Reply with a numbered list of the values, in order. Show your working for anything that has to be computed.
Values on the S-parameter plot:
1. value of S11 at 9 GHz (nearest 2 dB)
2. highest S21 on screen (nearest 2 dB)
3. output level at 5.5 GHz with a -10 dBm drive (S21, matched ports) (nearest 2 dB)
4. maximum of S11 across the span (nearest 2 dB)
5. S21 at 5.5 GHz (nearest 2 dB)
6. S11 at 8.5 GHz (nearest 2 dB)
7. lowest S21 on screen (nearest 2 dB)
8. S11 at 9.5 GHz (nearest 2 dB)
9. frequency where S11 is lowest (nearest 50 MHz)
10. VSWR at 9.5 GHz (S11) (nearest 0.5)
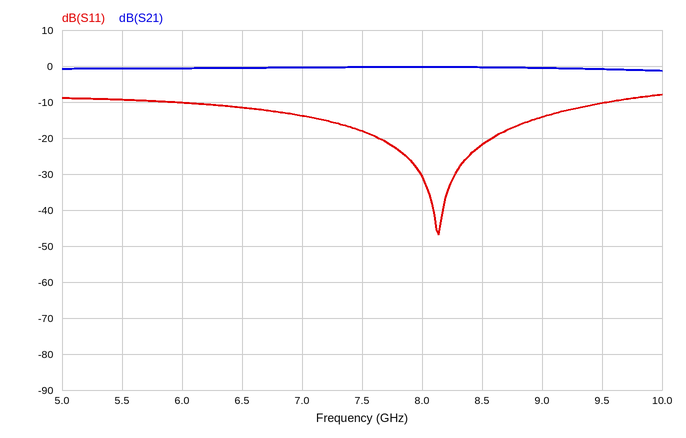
1. -14 dB
2. 0 dB
3. -10 dBm + (0 dB) = -10 dBm
4. -8 dB
5. 0 dB
6. -22 dB
7. -2 dB
8. -10 dB
9. 8.15 GHz
10. |Γ| = 10^(-10/20) = 0.3162; VSWR = (1 + 0.3162)/(1 − 0.3162) ≈ 1.92, so 2.0 to the nearest 0.5
